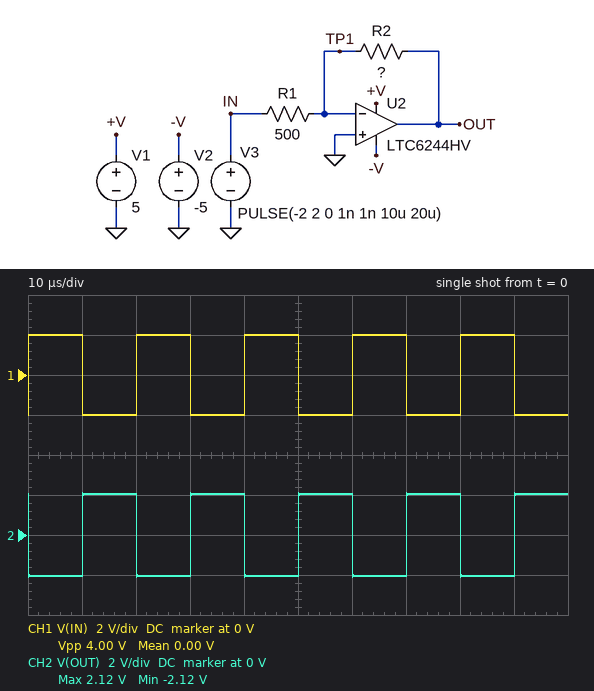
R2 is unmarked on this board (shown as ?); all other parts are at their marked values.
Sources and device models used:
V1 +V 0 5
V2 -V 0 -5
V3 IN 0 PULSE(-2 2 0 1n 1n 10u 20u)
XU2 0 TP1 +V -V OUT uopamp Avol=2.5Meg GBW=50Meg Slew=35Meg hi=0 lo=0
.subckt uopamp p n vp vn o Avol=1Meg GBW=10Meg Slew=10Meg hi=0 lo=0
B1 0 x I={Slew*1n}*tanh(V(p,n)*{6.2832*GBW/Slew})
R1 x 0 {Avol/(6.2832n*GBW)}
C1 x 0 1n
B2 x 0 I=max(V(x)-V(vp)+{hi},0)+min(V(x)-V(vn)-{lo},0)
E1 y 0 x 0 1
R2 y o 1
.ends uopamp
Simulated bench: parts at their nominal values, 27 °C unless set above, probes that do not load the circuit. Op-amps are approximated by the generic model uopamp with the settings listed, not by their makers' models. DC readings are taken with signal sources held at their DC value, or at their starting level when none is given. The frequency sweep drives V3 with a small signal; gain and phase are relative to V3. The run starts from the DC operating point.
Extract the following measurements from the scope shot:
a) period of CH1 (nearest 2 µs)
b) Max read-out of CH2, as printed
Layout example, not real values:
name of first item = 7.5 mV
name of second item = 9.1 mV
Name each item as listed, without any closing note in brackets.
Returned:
period of CH1 = 20 µs
Max read-out of CH2, as printed = 2.12 V
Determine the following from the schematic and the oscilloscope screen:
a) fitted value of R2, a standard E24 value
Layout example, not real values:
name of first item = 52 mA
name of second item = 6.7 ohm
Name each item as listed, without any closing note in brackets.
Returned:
fitted value of R2, a standard E24 value = 510 Ω
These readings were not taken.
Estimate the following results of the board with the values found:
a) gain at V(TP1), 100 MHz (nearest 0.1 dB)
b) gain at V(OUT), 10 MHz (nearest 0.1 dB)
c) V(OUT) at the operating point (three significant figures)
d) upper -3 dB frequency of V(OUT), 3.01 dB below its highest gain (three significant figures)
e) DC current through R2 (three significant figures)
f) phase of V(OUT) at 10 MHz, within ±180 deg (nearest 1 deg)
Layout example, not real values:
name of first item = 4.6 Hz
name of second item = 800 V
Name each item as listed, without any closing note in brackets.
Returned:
gain at V(TP1), 100 MHz = -6.2 dB
gain at V(OUT), 10 MHz = -0.5 dB
V(OUT) at the operating point = 2.04 V
upper -3 dB frequency of V(OUT), 3.01 dB below its highest gain = 24.7 MHz
DC current through R2 = 4.00 mA
phase of V(OUT) at 10 MHz, within ±180 deg = 158 deg
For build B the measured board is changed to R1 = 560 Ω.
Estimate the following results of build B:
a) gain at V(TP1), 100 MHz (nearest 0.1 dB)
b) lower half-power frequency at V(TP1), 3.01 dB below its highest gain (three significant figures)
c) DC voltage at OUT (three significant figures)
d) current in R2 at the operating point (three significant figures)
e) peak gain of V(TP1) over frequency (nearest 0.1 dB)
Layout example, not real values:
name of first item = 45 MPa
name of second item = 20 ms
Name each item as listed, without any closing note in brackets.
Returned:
gain at V(TP1), 100 MHz = -6.7 dB
lower half-power frequency at V(TP1), 3.01 dB below its highest gain = 26.1 MHz
DC voltage at OUT = 1.82 V
current in R2 at the operating point = 3.57 mA
peak gain of V(TP1) over frequency = -6.4 dB
